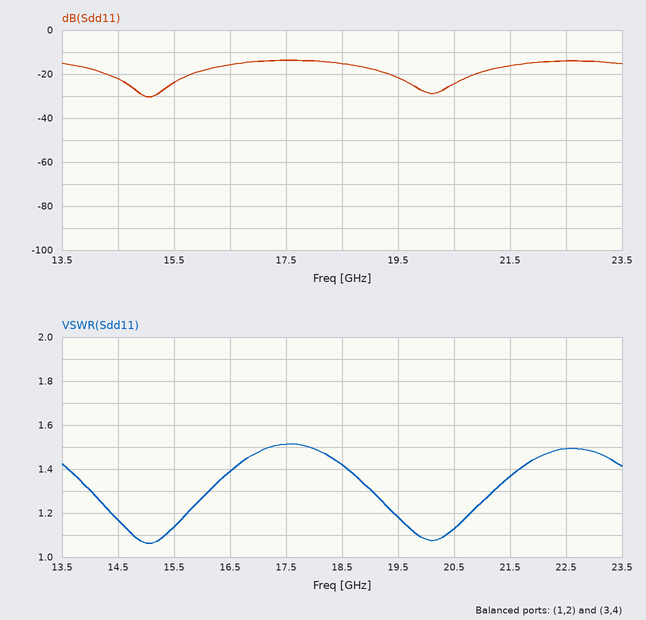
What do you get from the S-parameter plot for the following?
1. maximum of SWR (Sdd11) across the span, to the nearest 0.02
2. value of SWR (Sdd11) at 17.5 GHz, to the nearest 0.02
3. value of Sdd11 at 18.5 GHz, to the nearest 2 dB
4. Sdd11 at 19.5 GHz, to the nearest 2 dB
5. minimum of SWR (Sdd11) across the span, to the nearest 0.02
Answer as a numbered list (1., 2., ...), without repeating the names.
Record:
1. 1.52
2. 1.52
3. -16 dB
4. -22 dB
5. 1.06
